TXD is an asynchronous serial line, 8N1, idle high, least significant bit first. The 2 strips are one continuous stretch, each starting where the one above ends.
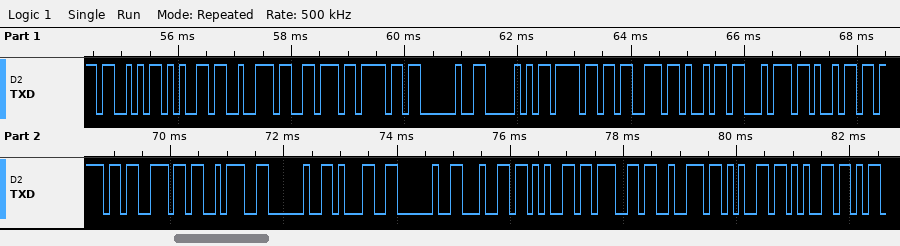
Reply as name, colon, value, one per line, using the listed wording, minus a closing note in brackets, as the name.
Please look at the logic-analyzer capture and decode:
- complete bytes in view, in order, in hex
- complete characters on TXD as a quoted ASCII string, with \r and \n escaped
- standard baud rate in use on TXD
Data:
complete bytes in view, in order, in hex: 53 65 72 76 6F 20 50 6F 73 69 74 69 6F 6E 3A 20 31 20 64 65 67 72 65 65
complete characters on TXD as a quoted ASCII string, with \r and \n escaped: "Servo Position: 1 degree"
standard baud rate in use on TXD: 9600 baud
